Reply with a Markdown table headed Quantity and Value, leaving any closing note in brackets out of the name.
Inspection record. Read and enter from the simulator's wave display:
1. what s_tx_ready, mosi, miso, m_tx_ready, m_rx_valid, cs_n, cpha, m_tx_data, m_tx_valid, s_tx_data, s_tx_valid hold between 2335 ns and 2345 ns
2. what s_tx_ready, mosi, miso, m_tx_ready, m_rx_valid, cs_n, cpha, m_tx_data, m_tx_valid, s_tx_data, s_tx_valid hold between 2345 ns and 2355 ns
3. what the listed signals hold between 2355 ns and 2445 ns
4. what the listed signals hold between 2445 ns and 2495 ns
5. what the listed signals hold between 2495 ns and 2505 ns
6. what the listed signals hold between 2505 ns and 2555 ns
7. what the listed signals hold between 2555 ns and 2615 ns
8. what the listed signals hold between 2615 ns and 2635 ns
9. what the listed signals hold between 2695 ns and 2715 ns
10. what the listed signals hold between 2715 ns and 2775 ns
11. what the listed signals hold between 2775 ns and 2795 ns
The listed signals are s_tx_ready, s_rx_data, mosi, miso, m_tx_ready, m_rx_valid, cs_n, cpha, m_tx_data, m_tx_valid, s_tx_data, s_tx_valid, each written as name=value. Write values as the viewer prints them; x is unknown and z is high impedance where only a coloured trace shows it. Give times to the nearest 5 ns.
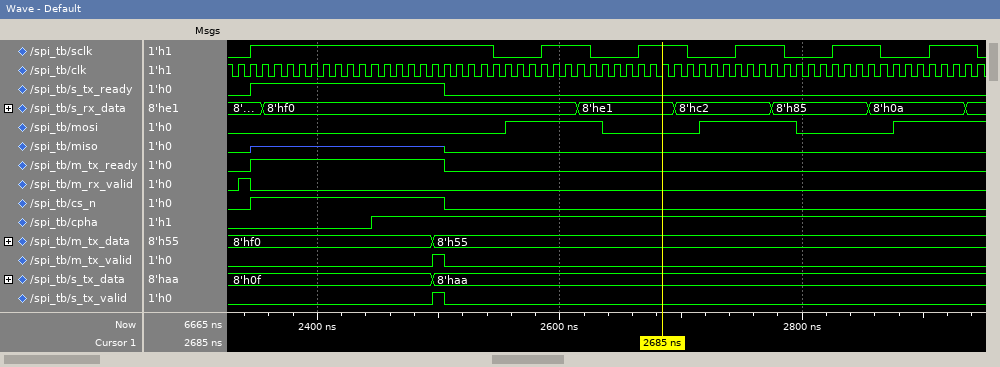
| Quantity | Value |
|---|---|
| what s_tx_ready, mosi, miso, m_tx_ready, m_rx_valid, cs_n, cpha, m_tx_data, m_tx_valid, s_tx_data, s_tx_valid hold between 2335 ns and 2345 ns | s_tx_ready=0, mosi=0, miso=0, m_tx_ready=0, m_rx_valid=1, cs_n=0, cpha=0, m_tx_data=8'hf0, m_tx_valid=0, s_tx_data=8'h0f, s_tx_valid=0 |
| what s_tx_ready, mosi, miso, m_tx_ready, m_rx_valid, cs_n, cpha, m_tx_data, m_tx_valid, s_tx_data, s_tx_valid hold between 2345 ns and 2355 ns | s_tx_ready=1, mosi=0, miso=z, m_tx_ready=1, m_rx_valid=0, cs_n=1, cpha=0, m_tx_data=8'hf0, m_tx_valid=0, s_tx_data=8'h0f, s_tx_valid=0 |
| what the listed signals hold between 2355 ns and 2445 ns | s_tx_ready=1, s_rx_data=8'hf0, mosi=0, miso=z, m_tx_ready=1, m_rx_valid=0, cs_n=1, cpha=0, m_tx_data=8'hf0, m_tx_valid=0, s_tx_data=8'h0f, s_tx_valid=0 |
| what the listed signals hold between 2445 ns and 2495 ns | s_tx_ready=1, s_rx_data=8'hf0, mosi=0, miso=z, m_tx_ready=1, m_rx_valid=0, cs_n=1, cpha=1, m_tx_data=8'hf0, m_tx_valid=0, s_tx_data=8'h0f, s_tx_valid=0 |
| what the listed signals hold between 2495 ns and 2505 ns | s_tx_ready=1, s_rx_data=8'hf0, mosi=0, miso=z, m_tx_ready=1, m_rx_valid=0, cs_n=1, cpha=1, m_tx_data=8'h55, m_tx_valid=1, s_tx_data=8'haa, s_tx_valid=1 |
| what the listed signals hold between 2505 ns and 2555 ns | s_tx_ready=0, s_rx_data=8'hf0, mosi=0, miso=0, m_tx_ready=0, m_rx_valid=0, cs_n=0, cpha=1, m_tx_data=8'h55, m_tx_valid=0, s_tx_data=8'haa, s_tx_valid=0 |
| what the listed signals hold between 2555 ns and 2615 ns | s_tx_ready=0, s_rx_data=8'hf0, mosi=1, miso=0, m_tx_ready=0, m_rx_valid=0, cs_n=0, cpha=1, m_tx_data=8'h55, m_tx_valid=0, s_tx_data=8'haa, s_tx_valid=0 |
| what the listed signals hold between 2615 ns and 2635 ns | s_tx_ready=0, s_rx_data=8'he1, mosi=1, miso=0, m_tx_ready=0, m_rx_valid=0, cs_n=0, cpha=1, m_tx_data=8'h55, m_tx_valid=0, s_tx_data=8'haa, s_tx_valid=0 |
| what the listed signals hold between 2695 ns and 2715 ns | s_tx_ready=0, s_rx_data=8'hc2, mosi=0, miso=0, m_tx_ready=0, m_rx_valid=0, cs_n=0, cpha=1, m_tx_data=8'h55, m_tx_valid=0, s_tx_data=8'haa, s_tx_valid=0 |
| what the listed signals hold between 2715 ns and 2775 ns | s_tx_ready=0, s_rx_data=8'hc2, mosi=1, miso=0, m_tx_ready=0, m_rx_valid=0, cs_n=0, cpha=1, m_tx_data=8'h55, m_tx_valid=0, s_tx_data=8'haa, s_tx_valid=0 |
| what the listed signals hold between 2775 ns and 2795 ns | s_tx_ready=0, s_rx_data=8'h85, mosi=1, miso=0, m_tx_ready=0, m_rx_valid=0, cs_n=0, cpha=1, m_tx_data=8'h55, m_tx_valid=0, s_tx_data=8'haa, s_tx_valid=0 |
